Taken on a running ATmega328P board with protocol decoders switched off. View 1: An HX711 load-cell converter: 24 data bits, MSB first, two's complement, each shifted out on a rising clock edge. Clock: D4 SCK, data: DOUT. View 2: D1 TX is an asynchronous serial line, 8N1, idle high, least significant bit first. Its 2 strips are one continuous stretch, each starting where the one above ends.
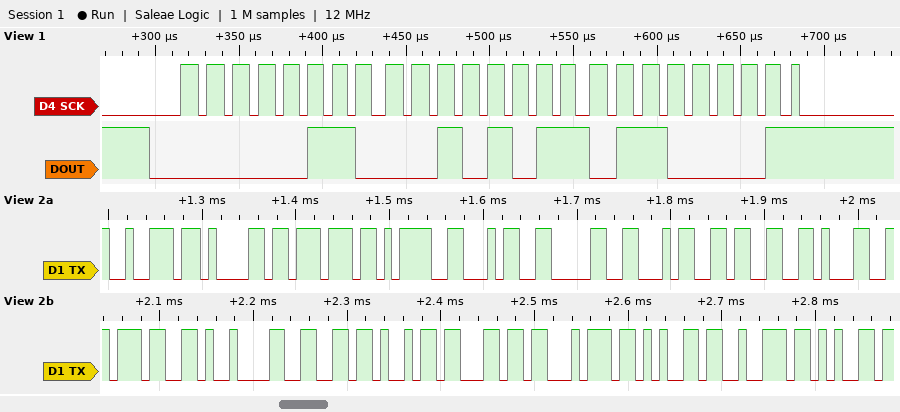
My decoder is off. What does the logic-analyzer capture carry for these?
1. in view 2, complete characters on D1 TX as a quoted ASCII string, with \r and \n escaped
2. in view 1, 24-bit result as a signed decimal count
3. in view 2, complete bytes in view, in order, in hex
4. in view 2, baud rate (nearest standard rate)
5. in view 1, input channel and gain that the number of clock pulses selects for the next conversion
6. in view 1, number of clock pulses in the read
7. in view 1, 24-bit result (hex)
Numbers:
"raw=404317\tfiltere"
404321
72 61 77 3D 34 30 34 33 31 37 09 66 69 6C 74 65 72 65
115200 baud
channel A, gain 128
25
0x062B61
